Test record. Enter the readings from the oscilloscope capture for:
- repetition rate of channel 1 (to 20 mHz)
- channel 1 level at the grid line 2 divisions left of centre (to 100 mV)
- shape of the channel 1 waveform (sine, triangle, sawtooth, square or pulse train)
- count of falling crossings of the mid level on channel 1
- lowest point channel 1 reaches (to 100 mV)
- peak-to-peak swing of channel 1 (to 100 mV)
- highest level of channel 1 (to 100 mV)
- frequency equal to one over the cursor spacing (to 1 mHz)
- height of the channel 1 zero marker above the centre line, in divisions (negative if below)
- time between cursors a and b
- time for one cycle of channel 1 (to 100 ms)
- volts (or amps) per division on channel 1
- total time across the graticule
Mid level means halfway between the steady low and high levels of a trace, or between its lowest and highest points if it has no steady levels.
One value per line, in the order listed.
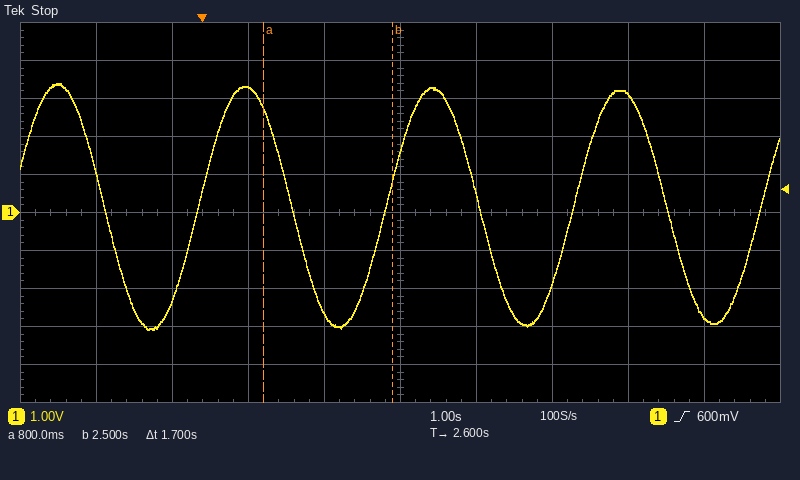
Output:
400 mHz
3.3 V
sine
4
-3.1 V
6.5 V
3.4 V
588 mHz
0.0 div
1.7 s
2.5 s
1 V
10 s
